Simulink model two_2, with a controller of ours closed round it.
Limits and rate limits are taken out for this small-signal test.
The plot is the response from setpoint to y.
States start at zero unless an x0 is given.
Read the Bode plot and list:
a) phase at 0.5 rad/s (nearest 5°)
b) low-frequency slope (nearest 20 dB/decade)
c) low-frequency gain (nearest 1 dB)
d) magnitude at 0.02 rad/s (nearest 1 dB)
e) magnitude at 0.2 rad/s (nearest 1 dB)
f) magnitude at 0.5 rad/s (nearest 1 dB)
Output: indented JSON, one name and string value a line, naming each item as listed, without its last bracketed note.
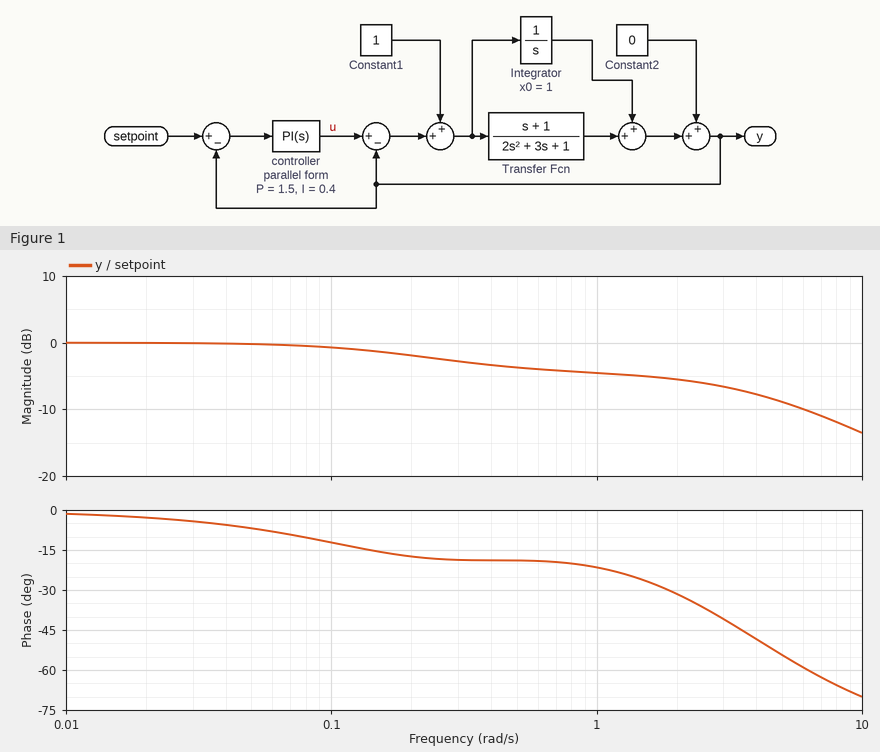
{
  "phase at 0.5 rad/s": "-20°",
  "low-frequency slope": "0 dB/decade",
  "low-frequency gain": "0 dB",
  "magnitude at 0.02 rad/s": "0 dB",
  "magnitude at 0.2 rad/s": "-2 dB",
  "magnitude at 0.5 rad/s": "-4 dB"
}
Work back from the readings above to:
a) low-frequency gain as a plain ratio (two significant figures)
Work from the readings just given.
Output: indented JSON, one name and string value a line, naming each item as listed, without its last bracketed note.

{
  "low-frequency gain as a plain ratio": "1.0"
}
